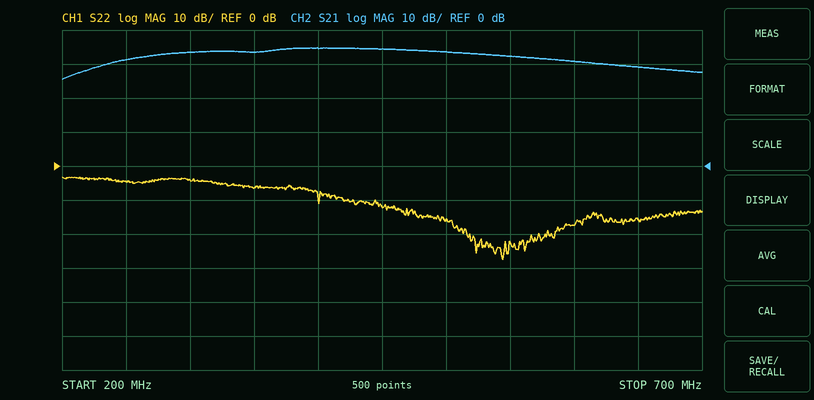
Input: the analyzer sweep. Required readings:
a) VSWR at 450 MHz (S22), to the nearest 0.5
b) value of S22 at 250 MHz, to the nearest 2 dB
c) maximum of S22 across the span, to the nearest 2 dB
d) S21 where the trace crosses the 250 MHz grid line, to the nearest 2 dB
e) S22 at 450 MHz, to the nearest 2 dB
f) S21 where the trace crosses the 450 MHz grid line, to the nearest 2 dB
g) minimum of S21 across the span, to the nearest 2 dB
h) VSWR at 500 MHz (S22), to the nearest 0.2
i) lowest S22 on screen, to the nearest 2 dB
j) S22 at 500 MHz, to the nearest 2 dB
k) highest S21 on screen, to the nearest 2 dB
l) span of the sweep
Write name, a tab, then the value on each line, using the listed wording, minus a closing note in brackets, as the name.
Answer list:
VSWR at 450 MHz (S22), to the nearest 0.5	1.5
value of S22 at 250 MHz, to the nearest 2 dB	-4 dB
maximum of S22 across the span, to the nearest 2 dB	-4 dB
S21 where the trace crosses the 250 MHz grid line, to the nearest 2 dB	32 dB
S22 at 450 MHz, to the nearest 2 dB	-12 dB
S21 where the trace crosses the 450 MHz grid line, to the nearest 2 dB	34 dB
minimum of S21 across the span, to the nearest 2 dB	26 dB
VSWR at 500 MHz (S22), to the nearest 0.2	1.4
lowest S22 on screen, to the nearest 2 dB	-28 dB
S22 at 500 MHz, to the nearest 2 dB	-16 dB
highest S21 on screen, to the nearest 2 dB	34 dB
span of the sweep	500 MHz
